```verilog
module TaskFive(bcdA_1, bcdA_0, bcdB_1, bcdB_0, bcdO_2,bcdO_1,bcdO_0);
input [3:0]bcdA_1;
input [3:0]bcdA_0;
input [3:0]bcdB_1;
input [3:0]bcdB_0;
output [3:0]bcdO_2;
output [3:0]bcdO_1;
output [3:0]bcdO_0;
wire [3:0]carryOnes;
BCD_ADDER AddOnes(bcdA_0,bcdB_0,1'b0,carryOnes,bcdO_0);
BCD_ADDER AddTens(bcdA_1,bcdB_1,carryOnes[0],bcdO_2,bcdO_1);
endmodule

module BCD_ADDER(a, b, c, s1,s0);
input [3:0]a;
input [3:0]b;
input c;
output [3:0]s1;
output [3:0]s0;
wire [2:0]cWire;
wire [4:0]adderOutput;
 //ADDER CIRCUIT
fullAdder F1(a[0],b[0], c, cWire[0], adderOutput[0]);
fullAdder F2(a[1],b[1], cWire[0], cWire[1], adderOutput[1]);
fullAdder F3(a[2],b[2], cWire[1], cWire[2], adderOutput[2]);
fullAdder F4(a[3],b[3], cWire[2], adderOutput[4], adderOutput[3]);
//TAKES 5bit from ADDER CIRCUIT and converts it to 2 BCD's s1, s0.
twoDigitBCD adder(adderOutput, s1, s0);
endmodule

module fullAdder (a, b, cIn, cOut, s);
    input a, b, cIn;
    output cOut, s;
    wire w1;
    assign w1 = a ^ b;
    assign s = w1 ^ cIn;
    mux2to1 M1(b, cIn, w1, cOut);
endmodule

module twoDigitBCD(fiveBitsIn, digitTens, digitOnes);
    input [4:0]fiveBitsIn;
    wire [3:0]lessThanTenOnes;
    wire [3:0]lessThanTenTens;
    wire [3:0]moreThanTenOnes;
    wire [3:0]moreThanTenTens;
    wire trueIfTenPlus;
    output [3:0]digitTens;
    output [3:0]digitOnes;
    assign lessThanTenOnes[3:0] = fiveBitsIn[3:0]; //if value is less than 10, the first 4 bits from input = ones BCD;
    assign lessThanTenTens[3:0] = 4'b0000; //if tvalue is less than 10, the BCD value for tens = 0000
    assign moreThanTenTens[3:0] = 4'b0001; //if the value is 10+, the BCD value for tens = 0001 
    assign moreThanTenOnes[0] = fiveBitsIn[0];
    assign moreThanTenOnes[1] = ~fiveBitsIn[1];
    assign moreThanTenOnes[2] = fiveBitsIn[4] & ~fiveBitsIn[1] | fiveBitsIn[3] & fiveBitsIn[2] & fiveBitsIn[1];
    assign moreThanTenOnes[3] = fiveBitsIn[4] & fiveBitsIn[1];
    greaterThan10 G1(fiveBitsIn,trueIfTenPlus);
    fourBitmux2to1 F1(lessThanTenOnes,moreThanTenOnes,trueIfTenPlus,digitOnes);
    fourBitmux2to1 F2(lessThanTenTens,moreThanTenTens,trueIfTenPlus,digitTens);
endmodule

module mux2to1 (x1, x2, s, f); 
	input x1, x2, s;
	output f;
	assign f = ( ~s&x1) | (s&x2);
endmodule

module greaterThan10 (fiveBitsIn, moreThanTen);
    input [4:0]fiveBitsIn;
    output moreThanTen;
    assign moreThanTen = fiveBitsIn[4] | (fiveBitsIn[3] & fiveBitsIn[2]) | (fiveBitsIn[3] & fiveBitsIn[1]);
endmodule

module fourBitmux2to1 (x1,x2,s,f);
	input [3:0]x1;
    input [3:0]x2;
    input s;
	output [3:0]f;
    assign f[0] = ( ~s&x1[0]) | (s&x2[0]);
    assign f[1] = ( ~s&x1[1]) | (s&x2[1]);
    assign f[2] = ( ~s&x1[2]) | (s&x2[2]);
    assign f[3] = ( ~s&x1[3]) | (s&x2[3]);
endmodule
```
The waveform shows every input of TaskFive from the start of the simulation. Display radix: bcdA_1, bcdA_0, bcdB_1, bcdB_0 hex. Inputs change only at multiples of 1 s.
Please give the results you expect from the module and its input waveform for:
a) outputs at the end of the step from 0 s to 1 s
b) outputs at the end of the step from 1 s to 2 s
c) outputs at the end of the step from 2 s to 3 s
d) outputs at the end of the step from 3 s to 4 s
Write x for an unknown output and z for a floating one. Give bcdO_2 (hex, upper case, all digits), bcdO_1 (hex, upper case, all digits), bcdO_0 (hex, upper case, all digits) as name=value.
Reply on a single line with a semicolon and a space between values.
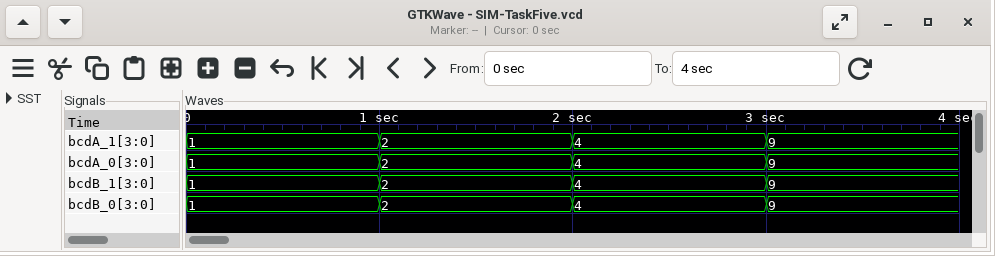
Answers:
bcdO_2=0, bcdO_1=2, bcdO_0=2; bcdO_2=0, bcdO_1=4, bcdO_0=4; bcdO_2=0, bcdO_1=8, bcdO_0=8; bcdO_2=1, bcdO_1=9, bcdO_0=8
